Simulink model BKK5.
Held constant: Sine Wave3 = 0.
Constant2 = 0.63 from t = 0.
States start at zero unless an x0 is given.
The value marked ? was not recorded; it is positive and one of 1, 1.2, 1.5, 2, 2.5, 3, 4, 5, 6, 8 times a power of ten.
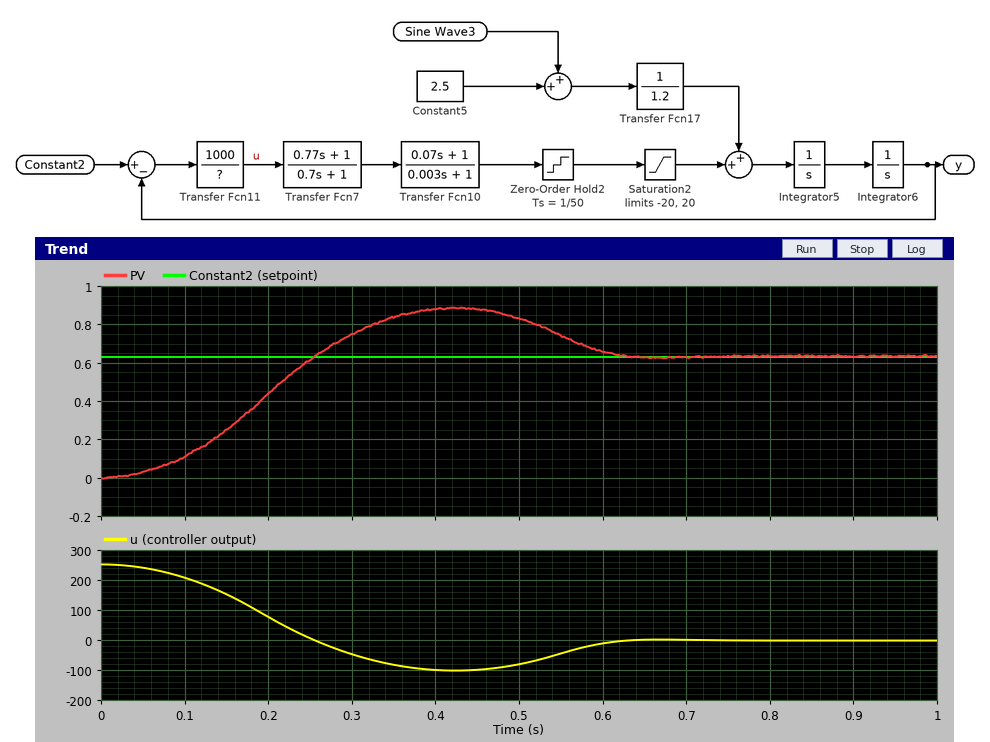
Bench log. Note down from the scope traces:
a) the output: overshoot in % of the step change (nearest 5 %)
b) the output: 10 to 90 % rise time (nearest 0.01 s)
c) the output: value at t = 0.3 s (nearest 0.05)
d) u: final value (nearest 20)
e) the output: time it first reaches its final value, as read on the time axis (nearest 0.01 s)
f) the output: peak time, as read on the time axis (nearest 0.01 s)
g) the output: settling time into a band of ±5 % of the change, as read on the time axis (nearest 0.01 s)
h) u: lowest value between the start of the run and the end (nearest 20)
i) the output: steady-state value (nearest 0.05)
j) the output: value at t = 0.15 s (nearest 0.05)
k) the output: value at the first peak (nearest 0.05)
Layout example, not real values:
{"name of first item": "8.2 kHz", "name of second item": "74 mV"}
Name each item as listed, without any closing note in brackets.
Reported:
{"the output: overshoot in % of the step change": "40 %", "the output: 10 to 90 % rise time": "0.16 s", "the output: value at t = 0.3 s": "0.75", "u: final value": "0", "the output: time it first reaches its final value, as read on the time axis": "0.26 s", "the output: peak time, as read on the time axis": "0.42 s", "the output: settling time into a band of ±5 % of the change, as read on the time axis": "0.59 s", "u: lowest value between the start of the run and the end": "-100", "the output: steady-state value": "0.65", "the output: value at t = 0.15 s": "0.25", "the output: value at the first peak": "0.90"}
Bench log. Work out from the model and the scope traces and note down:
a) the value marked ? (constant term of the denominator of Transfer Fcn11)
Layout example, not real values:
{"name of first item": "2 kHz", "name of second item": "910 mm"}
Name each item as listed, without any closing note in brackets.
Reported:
{"the value marked ?": "2.5"}
